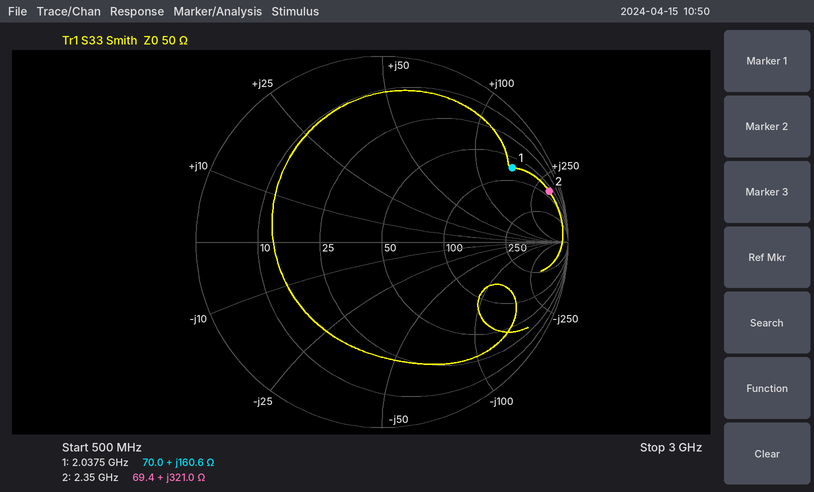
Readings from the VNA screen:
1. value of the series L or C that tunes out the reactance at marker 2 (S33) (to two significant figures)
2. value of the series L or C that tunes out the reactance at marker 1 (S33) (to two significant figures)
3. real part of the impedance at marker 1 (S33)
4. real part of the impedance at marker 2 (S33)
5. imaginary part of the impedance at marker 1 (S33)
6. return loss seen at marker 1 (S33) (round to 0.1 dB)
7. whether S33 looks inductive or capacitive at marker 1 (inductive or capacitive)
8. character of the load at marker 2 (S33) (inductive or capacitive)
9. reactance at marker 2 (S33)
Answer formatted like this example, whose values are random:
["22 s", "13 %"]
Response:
["210 fF", "490 fF", "70.0 Ω", "69.4 Ω", "+160.6 Ω", "1.9 dB", "inductive", "inductive", "+321.0 Ω"]
